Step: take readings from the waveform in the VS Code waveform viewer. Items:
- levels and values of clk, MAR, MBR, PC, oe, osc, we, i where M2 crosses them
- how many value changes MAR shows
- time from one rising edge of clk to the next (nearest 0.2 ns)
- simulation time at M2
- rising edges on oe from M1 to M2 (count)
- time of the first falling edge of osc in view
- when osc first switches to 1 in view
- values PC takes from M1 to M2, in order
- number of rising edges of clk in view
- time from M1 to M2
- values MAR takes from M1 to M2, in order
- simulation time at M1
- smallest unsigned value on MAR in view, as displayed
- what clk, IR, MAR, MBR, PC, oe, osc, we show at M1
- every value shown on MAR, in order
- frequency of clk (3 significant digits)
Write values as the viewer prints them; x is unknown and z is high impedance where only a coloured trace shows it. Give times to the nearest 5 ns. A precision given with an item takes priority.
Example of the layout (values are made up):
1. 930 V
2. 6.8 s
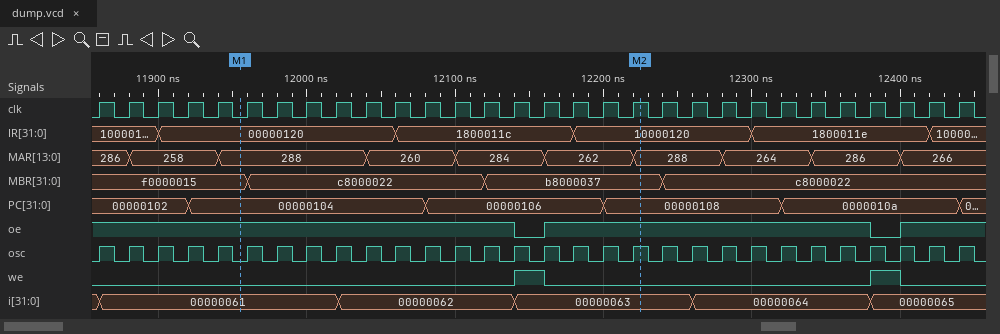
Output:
1. clk=1, MAR=288, MBR=b8000037, PC=00000108, oe=1, osc=1, we=0, i=00000063
2. 9
3. 20 ns
4. 12225 ns
5. 1
6. 11870 ns
7. 11860 ns
8. 00000104, 00000106, 00000108
9. 30
10. 270 ns
11. 288, 260, 284, 262, 288
12. 11955 ns
13. 258
14. clk=0, IR=00000120, MAR=288, MBR=f0000015, PC=00000104, oe=1, osc=0, we=0
15. 286, 258, 288, 260, 284, 262, 288, 264, 286, 266
16. 50.0 MHz
